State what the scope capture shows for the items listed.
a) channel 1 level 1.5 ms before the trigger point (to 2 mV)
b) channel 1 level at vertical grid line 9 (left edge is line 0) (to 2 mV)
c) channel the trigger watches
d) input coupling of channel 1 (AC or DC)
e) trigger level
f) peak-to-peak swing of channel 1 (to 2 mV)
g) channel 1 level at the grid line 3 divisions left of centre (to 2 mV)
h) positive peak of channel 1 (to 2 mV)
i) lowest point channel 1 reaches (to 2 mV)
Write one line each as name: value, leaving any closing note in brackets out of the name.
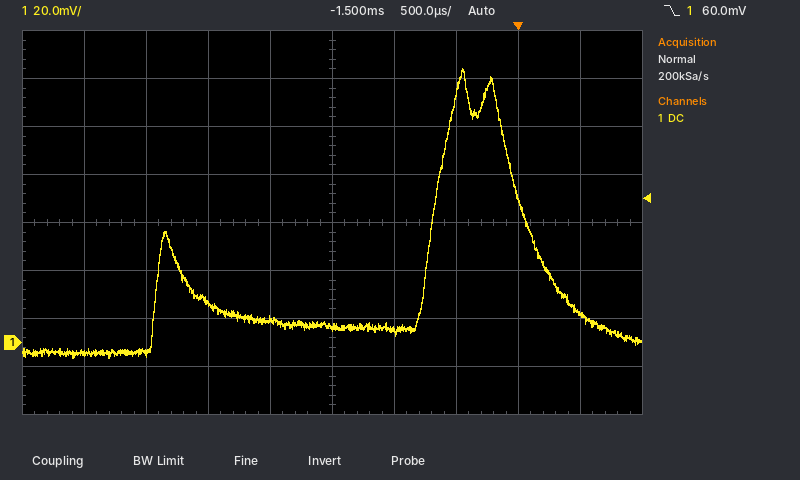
channel 1 level 1.5 ms before the trigger point: 6 mV
channel 1 level at vertical grid line 9 (left edge is line 0): 12 mV
channel the trigger watches: channel 1
input coupling of channel 1: DC
trigger level: 60.0 mV
peak-to-peak swing of channel 1: 120 mV
channel 1 level at the grid line 3 divisions left of centre: -4 mV
positive peak of channel 1: 114 mV
lowest point channel 1 reaches: -6 mV
